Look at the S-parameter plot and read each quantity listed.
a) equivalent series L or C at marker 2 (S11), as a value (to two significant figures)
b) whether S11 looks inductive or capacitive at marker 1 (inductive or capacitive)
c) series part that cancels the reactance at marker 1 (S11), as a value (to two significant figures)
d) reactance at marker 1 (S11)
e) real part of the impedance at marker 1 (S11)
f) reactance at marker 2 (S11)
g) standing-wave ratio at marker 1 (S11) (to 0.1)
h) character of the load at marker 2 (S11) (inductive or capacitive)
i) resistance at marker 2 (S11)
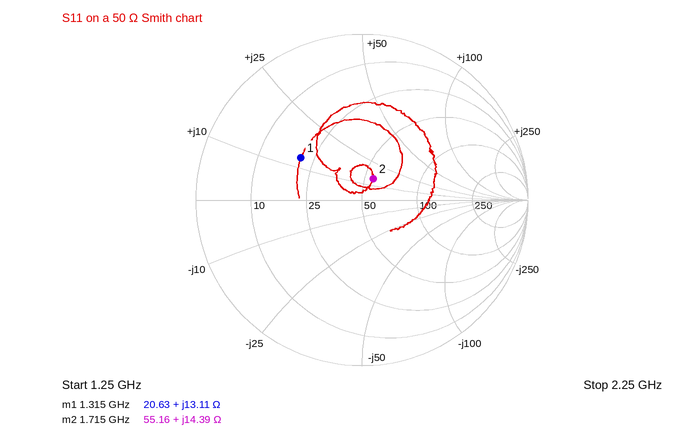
1.3 nH
inductive
9.2 pF
+13.11 Ω
20.63 Ω
+14.39 Ω
2.6
inductive
55.16 Ω
